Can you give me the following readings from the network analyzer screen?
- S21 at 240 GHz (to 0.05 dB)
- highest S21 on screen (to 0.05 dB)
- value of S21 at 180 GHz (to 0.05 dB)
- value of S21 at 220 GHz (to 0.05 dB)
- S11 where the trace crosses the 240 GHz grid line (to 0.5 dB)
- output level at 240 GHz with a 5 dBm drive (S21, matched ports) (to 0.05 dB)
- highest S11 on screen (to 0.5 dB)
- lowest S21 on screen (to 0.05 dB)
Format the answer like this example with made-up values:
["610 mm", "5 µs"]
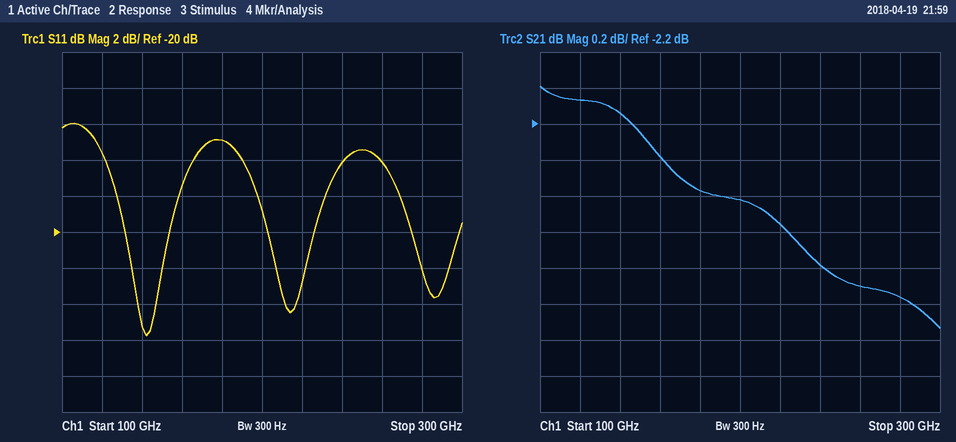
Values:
["-3.00 dB", "-2.00 dB", "-2.55 dB", "-2.75 dB", "-16.0 dB", "2.00 dBm", "-14.0 dB", "-3.35 dB"]
